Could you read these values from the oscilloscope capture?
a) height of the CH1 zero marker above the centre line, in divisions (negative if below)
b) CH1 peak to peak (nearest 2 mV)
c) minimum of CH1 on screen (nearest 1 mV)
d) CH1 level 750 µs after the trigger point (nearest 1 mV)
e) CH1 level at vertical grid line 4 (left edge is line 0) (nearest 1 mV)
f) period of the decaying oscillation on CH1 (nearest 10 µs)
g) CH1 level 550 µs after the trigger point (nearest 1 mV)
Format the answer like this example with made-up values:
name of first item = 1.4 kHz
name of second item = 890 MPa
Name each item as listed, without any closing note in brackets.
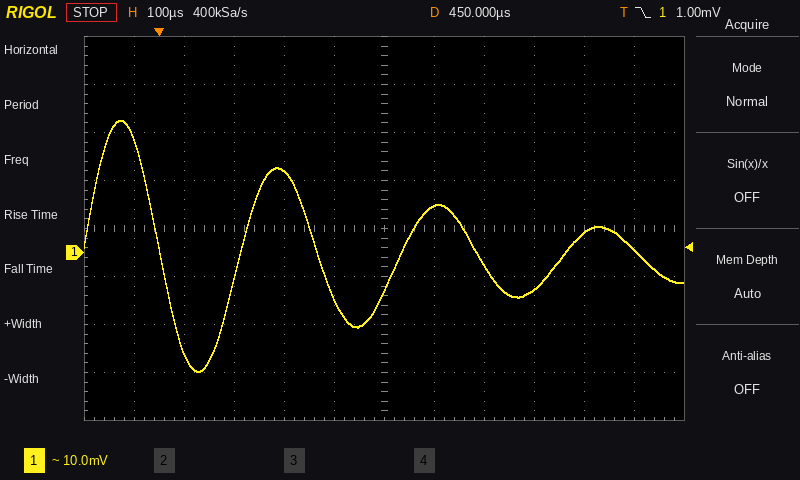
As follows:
height of the CH1 zero marker above the centre line, in divisions = -0.5 div
CH1 peak to peak = 52 mV
minimum of CH1 on screen = -25 mV
CH1 level 750 µs after the trigger point = -8 mV
CH1 level at vertical grid line 4 (left edge is line 0) = 17 mV
period of the decaying oscillation on CH1 = 320 µs
CH1 level 550 µs after the trigger point = 10 mV
